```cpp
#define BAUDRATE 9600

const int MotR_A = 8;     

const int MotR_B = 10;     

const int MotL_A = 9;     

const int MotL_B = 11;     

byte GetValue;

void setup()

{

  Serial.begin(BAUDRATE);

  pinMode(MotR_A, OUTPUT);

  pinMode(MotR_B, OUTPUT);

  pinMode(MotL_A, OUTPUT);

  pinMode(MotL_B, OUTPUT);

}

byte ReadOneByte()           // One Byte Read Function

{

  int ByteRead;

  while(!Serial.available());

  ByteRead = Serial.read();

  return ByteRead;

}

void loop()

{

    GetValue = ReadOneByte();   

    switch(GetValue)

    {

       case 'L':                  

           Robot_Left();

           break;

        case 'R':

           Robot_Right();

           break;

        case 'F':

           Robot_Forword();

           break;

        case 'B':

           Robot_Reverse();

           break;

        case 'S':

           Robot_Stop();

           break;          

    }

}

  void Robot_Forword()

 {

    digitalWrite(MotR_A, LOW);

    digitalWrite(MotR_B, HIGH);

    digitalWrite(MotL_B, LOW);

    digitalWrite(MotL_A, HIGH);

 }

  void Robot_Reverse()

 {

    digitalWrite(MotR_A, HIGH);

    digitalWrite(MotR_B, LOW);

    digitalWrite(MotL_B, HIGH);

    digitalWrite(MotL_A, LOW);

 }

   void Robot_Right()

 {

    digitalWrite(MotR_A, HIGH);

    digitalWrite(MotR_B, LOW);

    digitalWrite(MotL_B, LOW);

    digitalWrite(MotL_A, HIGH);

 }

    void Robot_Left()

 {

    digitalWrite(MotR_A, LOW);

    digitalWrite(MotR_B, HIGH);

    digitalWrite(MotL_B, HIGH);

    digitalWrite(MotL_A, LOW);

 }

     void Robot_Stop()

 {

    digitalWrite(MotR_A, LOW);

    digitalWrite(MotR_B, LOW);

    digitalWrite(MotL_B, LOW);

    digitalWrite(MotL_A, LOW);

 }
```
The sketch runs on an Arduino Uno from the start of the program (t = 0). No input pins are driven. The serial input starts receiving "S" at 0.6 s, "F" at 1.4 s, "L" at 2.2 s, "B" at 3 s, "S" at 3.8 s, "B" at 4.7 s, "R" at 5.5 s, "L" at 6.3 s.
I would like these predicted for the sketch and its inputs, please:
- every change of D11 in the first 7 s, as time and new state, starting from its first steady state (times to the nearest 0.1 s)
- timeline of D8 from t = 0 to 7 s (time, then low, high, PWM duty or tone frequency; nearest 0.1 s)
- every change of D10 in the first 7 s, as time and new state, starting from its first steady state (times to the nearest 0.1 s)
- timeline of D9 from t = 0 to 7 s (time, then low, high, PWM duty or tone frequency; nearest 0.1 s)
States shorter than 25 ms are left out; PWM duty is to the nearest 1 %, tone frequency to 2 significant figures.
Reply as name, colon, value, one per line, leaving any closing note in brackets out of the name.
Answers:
every change of D11 in the first 7 s, as time and new state, starting from its first steady state: 0 s low; 2.2 s high; 3.8 s low; 4.7 s high; 5.5 s low; 6.3 s high
timeline of D8 from t = 0 to 7 s: 0 s low; 3 s high; 3.8 s low; 4.7 s high; 6.3 s low
every change of D10 in the first 7 s, as time and new state, starting from its first steady state: 0 s low; 1.4 s high; 3 s low; 6.3 s high
timeline of D9 from t = 0 to 7 s: 0 s low; 1.4 s high; 2.2 s low; 5.5 s high; 6.3 s low
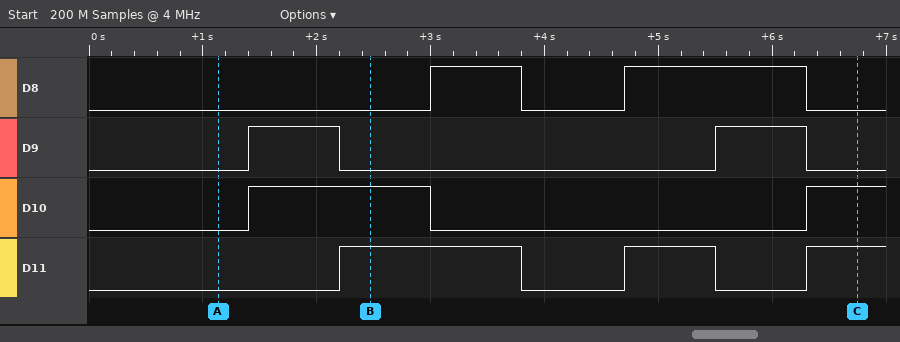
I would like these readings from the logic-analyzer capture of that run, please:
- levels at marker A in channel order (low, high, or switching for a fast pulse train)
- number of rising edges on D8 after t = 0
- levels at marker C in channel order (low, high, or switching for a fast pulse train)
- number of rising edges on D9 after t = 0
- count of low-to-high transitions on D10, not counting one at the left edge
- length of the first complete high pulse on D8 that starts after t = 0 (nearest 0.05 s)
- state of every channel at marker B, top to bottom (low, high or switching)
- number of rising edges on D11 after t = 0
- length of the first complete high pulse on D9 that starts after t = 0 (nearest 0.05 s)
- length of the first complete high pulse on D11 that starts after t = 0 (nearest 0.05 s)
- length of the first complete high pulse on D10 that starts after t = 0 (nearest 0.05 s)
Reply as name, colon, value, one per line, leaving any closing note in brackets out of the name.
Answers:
levels at marker A in channel order: D8 low, D9 low, D10 low, D11 low
number of rising edges on D8 after t = 0: 2
levels at marker C in channel order: D8 low, D9 low, D10 high, D11 high
number of rising edges on D9 after t = 0: 2
count of low-to-high transitions on D10, not counting one at the left edge: 2
length of the first complete high pulse on D8 that starts after t = 0: 0.80 s
state of every channel at marker B, top to bottom: D8 low, D9 low, D10 high, D11 high
number of rising edges on D11 after t = 0: 3
length of the first complete high pulse on D9 that starts after t = 0: 0.80 s
length of the first complete high pulse on D11 that starts after t = 0: 1.60 s
length of the first complete high pulse on D10 that starts after t = 0: 1.60 s
